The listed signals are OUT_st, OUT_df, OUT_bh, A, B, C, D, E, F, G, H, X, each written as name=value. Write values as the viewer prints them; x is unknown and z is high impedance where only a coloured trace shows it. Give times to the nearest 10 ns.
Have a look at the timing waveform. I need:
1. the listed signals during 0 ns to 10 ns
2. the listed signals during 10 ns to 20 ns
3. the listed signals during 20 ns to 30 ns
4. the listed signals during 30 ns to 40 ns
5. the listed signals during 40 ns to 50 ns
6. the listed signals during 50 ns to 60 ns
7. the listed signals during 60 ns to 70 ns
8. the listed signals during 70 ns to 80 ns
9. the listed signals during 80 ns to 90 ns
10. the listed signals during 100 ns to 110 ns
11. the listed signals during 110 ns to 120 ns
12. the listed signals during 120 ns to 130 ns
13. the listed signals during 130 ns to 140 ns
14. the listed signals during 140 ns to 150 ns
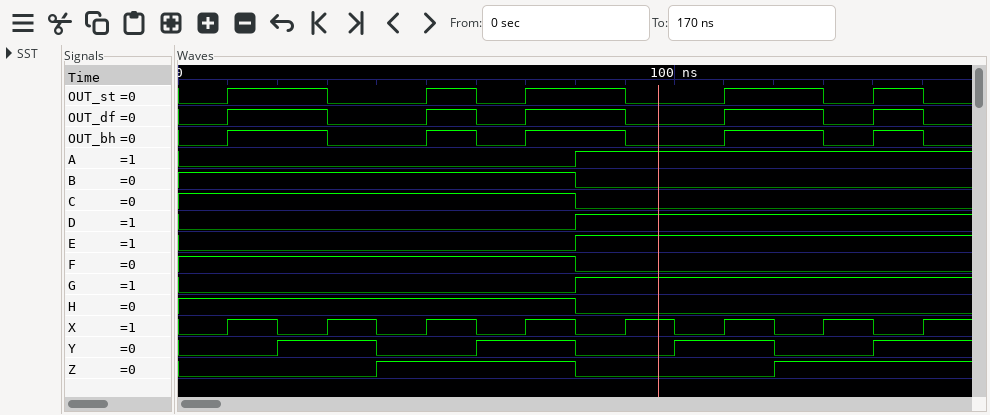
OUT_st=0, OUT_df=0, OUT_bh=0, A=0, B=1, C=1, D=0, E=0, F=1, G=0, H=1, X=0
OUT_st=1, OUT_df=1, OUT_bh=1, A=0, B=1, C=1, D=0, E=0, F=1, G=0, H=1, X=1
OUT_st=1, OUT_df=1, OUT_bh=1, A=0, B=1, C=1, D=0, E=0, F=1, G=0, H=1, X=0
OUT_st=0, OUT_df=0, OUT_bh=0, A=0, B=1, C=1, D=0, E=0, F=1, G=0, H=1, X=1
OUT_st=0, OUT_df=0, OUT_bh=0, A=0, B=1, C=1, D=0, E=0, F=1, G=0, H=1, X=0
OUT_st=1, OUT_df=1, OUT_bh=1, A=0, B=1, C=1, D=0, E=0, F=1, G=0, H=1, X=1
OUT_st=0, OUT_df=0, OUT_bh=0, A=0, B=1, C=1, D=0, E=0, F=1, G=0, H=1, X=0
OUT_st=1, OUT_df=1, OUT_bh=1, A=0, B=1, C=1, D=0, E=0, F=1, G=0, H=1, X=1
OUT_st=1, OUT_df=1, OUT_bh=1, A=1, B=0, C=0, D=1, E=1, F=0, G=1, H=0, X=0
OUT_st=0, OUT_df=0, OUT_bh=0, A=1, B=0, C=0, D=1, E=1, F=0, G=1, H=0, X=0
OUT_st=1, OUT_df=1, OUT_bh=1, A=1, B=0, C=0, D=1, E=1, F=0, G=1, H=0, X=1
OUT_st=1, OUT_df=1, OUT_bh=1, A=1, B=0, C=0, D=1, E=1, F=0, G=1, H=0, X=0
OUT_st=0, OUT_df=0, OUT_bh=0, A=1, B=0, C=0, D=1, E=1, F=0, G=1, H=0, X=1
OUT_st=1, OUT_df=1, OUT_bh=1, A=1, B=0, C=0, D=1, E=1, F=0, G=1, H=0, X=0
